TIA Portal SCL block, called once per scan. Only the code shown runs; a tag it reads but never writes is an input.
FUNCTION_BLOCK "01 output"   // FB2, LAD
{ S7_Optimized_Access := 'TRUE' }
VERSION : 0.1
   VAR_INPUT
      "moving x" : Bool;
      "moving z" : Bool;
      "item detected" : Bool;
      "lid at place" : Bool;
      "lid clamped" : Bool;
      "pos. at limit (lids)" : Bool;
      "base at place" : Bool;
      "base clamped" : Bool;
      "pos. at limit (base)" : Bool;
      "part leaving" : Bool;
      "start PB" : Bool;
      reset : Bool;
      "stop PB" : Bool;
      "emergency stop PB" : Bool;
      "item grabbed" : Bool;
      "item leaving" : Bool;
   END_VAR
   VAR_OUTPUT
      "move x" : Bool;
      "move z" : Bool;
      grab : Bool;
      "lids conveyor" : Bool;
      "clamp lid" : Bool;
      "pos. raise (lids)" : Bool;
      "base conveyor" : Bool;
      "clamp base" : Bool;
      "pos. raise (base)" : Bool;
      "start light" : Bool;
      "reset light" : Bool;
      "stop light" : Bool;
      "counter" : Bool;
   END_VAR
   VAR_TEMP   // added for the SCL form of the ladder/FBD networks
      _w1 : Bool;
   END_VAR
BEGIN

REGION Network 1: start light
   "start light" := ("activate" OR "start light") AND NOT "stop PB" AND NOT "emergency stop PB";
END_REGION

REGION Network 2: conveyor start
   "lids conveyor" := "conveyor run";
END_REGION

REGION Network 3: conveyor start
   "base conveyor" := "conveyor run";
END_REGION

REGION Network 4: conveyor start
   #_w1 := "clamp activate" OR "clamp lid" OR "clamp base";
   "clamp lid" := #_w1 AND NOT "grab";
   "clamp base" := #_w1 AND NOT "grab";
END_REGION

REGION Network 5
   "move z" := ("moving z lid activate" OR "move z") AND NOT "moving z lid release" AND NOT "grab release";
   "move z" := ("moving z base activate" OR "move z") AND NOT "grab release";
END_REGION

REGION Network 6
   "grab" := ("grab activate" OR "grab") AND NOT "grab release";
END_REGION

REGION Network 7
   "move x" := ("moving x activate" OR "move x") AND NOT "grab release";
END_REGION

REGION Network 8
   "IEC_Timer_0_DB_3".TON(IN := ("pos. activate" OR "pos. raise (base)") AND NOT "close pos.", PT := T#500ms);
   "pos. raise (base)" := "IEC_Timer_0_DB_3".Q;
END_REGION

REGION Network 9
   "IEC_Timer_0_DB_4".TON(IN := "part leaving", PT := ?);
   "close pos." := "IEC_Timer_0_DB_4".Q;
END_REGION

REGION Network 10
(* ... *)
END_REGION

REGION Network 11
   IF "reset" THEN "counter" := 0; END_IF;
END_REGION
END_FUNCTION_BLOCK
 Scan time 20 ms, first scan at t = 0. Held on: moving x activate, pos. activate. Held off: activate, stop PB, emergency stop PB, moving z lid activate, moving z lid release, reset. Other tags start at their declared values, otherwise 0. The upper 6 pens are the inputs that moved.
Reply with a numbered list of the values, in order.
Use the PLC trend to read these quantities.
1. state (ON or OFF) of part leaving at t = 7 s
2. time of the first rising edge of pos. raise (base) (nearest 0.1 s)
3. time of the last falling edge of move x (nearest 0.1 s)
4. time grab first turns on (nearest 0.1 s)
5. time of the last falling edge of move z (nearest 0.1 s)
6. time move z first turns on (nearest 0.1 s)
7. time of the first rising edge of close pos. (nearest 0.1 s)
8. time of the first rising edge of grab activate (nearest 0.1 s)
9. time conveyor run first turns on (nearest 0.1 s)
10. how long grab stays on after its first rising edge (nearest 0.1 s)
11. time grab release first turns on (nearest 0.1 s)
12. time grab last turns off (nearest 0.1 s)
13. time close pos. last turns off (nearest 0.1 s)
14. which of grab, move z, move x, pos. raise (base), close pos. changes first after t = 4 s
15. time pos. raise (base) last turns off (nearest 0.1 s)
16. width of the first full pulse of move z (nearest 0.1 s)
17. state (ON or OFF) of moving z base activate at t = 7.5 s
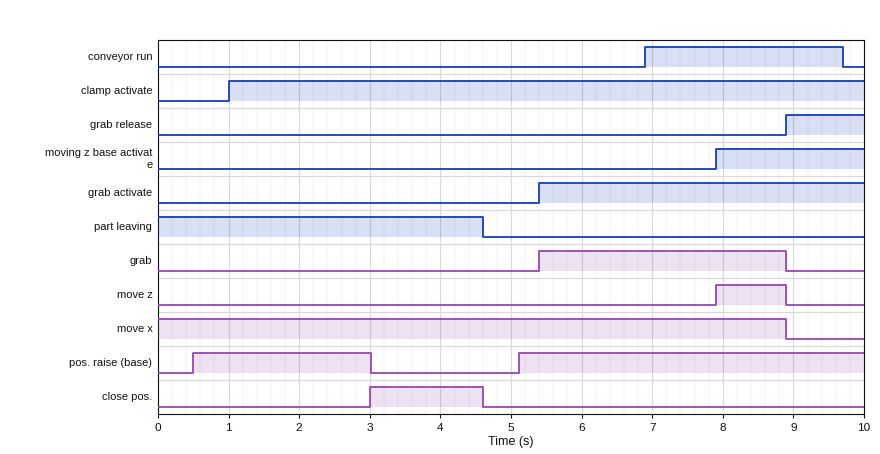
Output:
1. OFF
2. 0.5 s
3. 8.9 s
4. 5.4 s
5. 8.9 s
6. 7.9 s
7. 3.0 s
8. 5.4 s
9. 6.9 s
10. 3.5 s
11. 8.9 s
12. 8.9 s
13. 4.6 s
14. close pos.
15. 3.0 s
16. 1.0 s
17. OFF
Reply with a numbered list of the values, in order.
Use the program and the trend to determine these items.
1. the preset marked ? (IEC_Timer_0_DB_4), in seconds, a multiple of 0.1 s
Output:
1. 3.0 s
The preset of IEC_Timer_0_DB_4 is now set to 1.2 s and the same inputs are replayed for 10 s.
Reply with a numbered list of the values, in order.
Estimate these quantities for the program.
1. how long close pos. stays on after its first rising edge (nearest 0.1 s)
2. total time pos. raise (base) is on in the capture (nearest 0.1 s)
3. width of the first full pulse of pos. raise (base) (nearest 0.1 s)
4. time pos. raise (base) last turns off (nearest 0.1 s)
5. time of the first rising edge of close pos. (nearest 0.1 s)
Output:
1. 3.4 s
2. 5.6 s
3. 0.7 s
4. 1.2 s
5. 1.2 s
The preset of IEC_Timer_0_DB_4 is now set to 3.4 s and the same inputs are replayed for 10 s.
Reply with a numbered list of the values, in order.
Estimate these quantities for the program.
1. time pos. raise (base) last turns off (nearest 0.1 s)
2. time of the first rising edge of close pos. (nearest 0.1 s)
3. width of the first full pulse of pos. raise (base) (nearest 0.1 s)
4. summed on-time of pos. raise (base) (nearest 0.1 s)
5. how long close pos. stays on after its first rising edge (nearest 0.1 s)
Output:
1. 3.4 s
2. 3.4 s
3. 2.9 s
4. 7.8 s
5. 1.2 s
